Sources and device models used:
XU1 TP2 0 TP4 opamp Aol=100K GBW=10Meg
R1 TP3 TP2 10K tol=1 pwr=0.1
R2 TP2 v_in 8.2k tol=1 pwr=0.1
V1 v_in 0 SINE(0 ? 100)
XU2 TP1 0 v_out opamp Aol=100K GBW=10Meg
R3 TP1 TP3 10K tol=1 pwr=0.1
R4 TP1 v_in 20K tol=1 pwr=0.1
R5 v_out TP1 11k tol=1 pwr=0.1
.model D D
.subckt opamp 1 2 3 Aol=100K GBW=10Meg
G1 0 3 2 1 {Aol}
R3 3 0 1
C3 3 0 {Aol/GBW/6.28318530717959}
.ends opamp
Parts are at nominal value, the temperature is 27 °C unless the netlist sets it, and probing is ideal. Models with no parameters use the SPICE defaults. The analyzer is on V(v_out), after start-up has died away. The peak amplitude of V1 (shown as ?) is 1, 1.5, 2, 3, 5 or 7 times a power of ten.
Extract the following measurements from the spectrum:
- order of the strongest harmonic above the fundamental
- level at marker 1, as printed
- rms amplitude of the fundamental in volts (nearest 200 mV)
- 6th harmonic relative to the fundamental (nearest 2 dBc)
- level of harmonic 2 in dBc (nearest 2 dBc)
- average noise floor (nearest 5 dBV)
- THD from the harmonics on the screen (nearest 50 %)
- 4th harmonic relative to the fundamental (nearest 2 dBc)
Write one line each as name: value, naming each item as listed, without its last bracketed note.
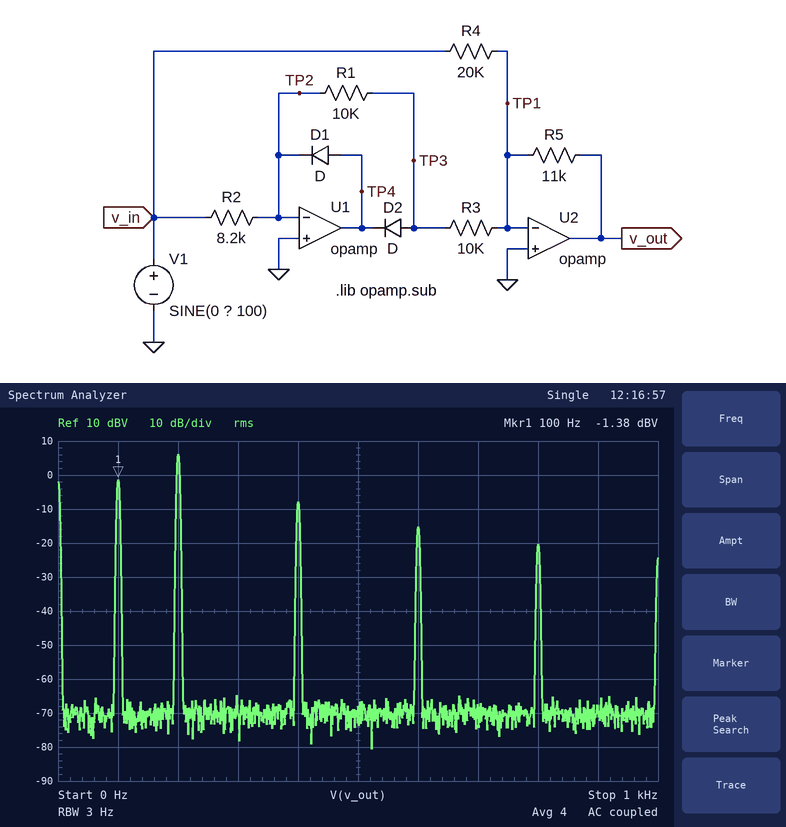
order of the strongest harmonic above the fundamental: 2
level at marker 1, as printed: -1.38 dBV
rms amplitude of the fundamental in volts: 800 mV
6th harmonic relative to the fundamental: -14 dBc
level of harmonic 2 in dBc: 8 dBc
average noise floor: -70 dBV
THD from the harmonics on the screen: 250 %
4th harmonic relative to the fundamental: -6 dBc
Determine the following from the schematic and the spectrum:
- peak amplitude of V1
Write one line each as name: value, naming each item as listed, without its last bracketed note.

peak amplitude of V1: 10 V
